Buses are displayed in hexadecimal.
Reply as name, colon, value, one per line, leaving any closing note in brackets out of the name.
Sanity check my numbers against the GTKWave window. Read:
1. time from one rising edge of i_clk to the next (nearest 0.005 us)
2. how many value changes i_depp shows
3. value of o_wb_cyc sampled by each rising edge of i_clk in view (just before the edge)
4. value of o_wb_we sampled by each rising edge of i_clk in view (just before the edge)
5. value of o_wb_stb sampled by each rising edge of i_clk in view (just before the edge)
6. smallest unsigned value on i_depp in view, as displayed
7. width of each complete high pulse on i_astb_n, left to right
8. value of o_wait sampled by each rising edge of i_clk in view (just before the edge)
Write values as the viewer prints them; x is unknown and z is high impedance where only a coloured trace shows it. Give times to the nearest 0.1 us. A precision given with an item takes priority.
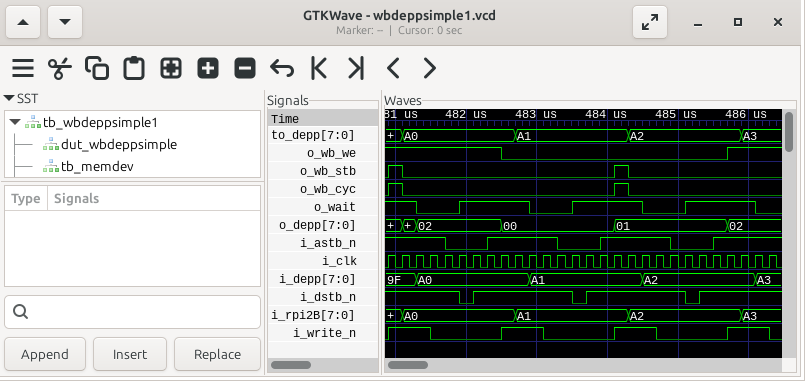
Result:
time from one rising edge of i_clk to the next: 0.2 us
how many value changes i_depp shows: 4
value of o_wb_cyc sampled by each rising edge of i_clk in view: 0 1 0 0 0 0 0 0 0 0 0 0 0 0 0 0 0 1 0 0 0 0 0 0 0 0 0 0
value of o_wb_we sampled by each rising edge of i_clk in view: 1 1 1 1 1 1 1 1 1 0 0 0 0 0 0 0 0 0 0 0 0 0 0 0 0 1 1 1
value of o_wb_stb sampled by each rising edge of i_clk in view: 0 1 0 0 0 0 0 0 0 0 0 0 0 0 0 0 0 1 0 0 0 0 0 0 0 0 0 0
smallest unsigned value on i_depp in view, as displayed: 9F
width of each complete high pulse on i_astb_n, left to right: 1 us, 1 us
value of o_wait sampled by each rising edge of i_clk in view: 1 1 1 0 0 0 1 1 1 1 1 0 0 0 1 1 1 1 1 0 0 0 1 1 1 1 1 0
